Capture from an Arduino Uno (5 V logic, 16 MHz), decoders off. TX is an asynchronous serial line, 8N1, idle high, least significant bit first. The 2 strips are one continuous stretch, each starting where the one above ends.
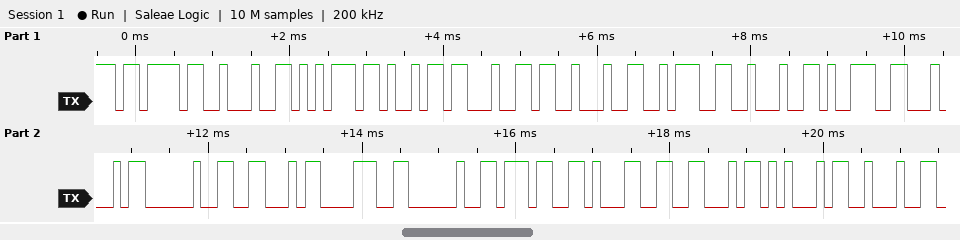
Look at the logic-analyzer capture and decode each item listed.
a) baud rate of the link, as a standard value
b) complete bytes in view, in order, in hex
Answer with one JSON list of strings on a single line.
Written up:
["9600 baud", "0x7B 0x22 0x75 0x69 0x64 0x22 0x3A 0x22 0x39 0x44 0x20 0x46 0x38 0x20 0x37 0x31 0x46 0x45 0x22"]
